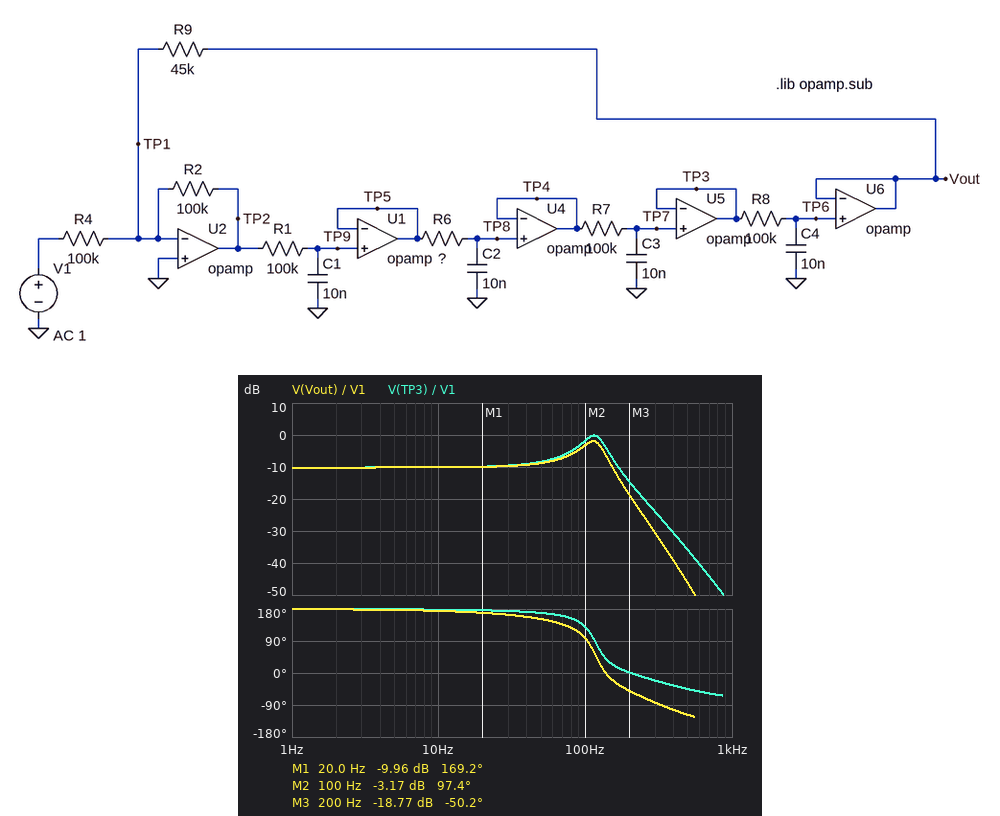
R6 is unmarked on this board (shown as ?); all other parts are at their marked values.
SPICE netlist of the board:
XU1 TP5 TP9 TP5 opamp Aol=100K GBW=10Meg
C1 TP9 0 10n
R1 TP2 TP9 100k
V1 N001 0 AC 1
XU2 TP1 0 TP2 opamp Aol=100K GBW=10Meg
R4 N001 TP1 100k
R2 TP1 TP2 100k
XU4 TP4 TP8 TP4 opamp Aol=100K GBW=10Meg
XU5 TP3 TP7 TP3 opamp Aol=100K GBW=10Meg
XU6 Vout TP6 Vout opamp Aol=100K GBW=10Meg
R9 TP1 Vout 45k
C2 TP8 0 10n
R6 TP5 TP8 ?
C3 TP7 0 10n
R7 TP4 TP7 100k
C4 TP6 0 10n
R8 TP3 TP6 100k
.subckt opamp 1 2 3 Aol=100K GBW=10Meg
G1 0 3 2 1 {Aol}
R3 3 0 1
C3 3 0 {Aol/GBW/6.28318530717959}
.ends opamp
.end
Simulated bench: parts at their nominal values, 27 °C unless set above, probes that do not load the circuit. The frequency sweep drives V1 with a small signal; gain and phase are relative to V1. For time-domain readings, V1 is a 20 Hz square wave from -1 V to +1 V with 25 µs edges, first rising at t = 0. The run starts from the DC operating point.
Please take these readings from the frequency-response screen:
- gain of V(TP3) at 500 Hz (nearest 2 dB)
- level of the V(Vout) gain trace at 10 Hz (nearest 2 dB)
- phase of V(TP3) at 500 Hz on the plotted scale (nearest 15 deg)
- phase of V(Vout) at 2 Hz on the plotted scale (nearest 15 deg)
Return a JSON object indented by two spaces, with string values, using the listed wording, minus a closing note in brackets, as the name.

{
  "gain of V(TP3) at 500 Hz": "-36 dB",
  "level of the V(Vout) gain trace at 10 Hz": "-10 dB",
  "phase of V(TP3) at 500 Hz on the plotted scale": "-45 deg",
  "phase of V(Vout) at 2 Hz on the plotted scale": "180 deg"
}
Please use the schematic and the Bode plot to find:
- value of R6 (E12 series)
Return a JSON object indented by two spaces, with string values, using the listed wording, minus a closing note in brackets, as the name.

{
  "value of R6": "180 kΩ"
}
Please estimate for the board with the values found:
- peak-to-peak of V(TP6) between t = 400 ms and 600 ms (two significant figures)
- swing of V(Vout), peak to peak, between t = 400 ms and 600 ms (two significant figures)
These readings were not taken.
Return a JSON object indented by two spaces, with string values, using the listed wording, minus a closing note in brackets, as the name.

{
  "peak-to-peak of V(TP6) between t = 400 ms and 600 ms": "1.2 V",
  "swing of V(Vout), peak to peak, between t = 400 ms and 600 ms": "1.2 V"
}
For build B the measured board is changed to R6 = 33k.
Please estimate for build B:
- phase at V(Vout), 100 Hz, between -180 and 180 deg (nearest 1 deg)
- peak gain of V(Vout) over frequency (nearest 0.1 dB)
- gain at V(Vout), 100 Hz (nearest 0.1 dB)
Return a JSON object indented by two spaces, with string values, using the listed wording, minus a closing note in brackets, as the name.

{
  "phase at V(Vout), 100 Hz, between -180 and 180 deg": "137 deg",
  "peak gain of V(Vout) over frequency": "-3.0 dB",
  "gain at V(Vout), 100 Hz": "-7.4 dB"
}
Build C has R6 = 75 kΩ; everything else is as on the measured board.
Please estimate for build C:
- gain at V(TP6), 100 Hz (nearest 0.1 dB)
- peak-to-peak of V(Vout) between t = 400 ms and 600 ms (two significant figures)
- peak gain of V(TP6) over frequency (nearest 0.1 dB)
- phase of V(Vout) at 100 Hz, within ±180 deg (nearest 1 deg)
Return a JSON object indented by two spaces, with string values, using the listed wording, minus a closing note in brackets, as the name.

{
  "gain at V(TP6), 100 Hz": "-6.0 dB",
  "peak-to-peak of V(Vout) between t = 400 ms and 600 ms": "1.3 V",
  "peak gain of V(TP6) over frequency": "-1.1 dB",
  "phase of V(Vout) at 100 Hz, within ±180 deg": "129 deg"
}
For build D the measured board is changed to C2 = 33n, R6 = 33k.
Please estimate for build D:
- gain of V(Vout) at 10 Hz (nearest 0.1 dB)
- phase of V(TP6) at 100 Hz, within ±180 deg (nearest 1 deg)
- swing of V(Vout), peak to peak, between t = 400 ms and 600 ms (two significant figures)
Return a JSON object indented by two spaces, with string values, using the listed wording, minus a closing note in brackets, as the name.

{
  "gain of V(Vout) at 10 Hz": "-10.1 dB",
  "phase of V(TP6) at 100 Hz, within ±180 deg": "121 deg",
  "swing of V(Vout), peak to peak, between t = 400 ms and 600 ms": "1.3 V"
}
